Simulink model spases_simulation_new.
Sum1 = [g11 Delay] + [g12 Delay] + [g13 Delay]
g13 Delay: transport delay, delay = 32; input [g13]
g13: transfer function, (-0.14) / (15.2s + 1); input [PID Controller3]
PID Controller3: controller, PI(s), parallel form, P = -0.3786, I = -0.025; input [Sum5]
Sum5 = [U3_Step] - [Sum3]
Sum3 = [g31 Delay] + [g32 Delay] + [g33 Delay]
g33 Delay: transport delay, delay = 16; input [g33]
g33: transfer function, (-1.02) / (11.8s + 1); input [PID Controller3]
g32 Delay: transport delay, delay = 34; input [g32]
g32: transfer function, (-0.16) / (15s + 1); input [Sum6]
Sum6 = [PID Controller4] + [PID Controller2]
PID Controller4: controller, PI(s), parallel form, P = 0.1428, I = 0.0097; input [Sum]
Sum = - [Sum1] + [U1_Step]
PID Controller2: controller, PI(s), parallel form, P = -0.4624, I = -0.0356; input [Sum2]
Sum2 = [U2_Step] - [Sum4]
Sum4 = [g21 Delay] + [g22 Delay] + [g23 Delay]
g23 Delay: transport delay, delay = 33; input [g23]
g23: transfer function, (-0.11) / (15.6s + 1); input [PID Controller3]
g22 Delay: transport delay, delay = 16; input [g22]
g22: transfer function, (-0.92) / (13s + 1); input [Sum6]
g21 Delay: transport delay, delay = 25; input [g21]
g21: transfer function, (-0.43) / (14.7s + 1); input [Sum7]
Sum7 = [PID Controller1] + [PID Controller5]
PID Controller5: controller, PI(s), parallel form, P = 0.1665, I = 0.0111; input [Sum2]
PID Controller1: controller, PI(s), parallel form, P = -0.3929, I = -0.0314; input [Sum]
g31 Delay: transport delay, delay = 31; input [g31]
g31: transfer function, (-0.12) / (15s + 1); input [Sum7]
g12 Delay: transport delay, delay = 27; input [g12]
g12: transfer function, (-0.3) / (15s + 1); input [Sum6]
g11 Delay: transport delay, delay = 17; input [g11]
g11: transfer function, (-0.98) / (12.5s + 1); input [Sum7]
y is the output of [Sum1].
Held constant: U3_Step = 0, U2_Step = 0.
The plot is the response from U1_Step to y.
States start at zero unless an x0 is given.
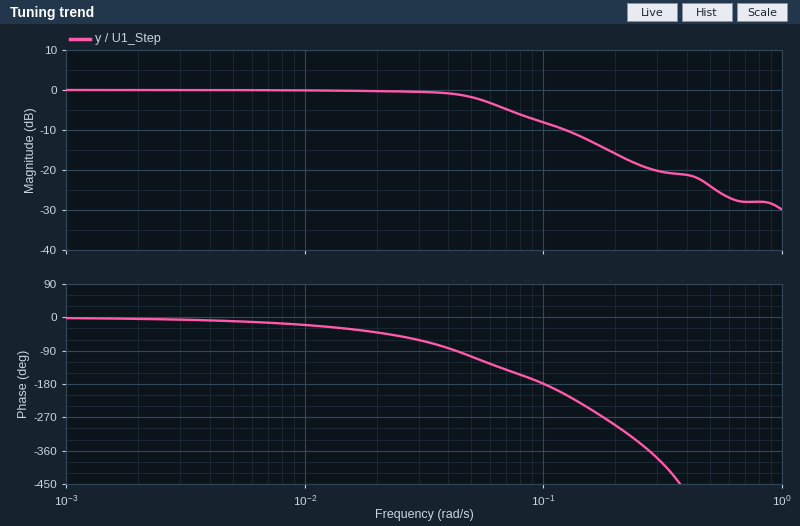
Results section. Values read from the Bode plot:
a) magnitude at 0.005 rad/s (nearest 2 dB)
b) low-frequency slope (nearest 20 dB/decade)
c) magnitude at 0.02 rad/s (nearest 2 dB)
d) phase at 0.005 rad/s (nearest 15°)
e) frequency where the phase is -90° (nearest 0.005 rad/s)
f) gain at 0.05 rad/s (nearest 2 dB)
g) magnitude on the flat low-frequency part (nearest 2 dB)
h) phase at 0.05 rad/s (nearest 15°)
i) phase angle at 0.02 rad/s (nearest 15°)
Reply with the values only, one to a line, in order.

0 dB
0 dB/decade
0 dB
-15°
0.045 rad/s
-2 dB
0 dB
-105°
-45°
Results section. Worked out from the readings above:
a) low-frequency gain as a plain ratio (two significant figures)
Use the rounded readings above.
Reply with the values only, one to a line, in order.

1.0
